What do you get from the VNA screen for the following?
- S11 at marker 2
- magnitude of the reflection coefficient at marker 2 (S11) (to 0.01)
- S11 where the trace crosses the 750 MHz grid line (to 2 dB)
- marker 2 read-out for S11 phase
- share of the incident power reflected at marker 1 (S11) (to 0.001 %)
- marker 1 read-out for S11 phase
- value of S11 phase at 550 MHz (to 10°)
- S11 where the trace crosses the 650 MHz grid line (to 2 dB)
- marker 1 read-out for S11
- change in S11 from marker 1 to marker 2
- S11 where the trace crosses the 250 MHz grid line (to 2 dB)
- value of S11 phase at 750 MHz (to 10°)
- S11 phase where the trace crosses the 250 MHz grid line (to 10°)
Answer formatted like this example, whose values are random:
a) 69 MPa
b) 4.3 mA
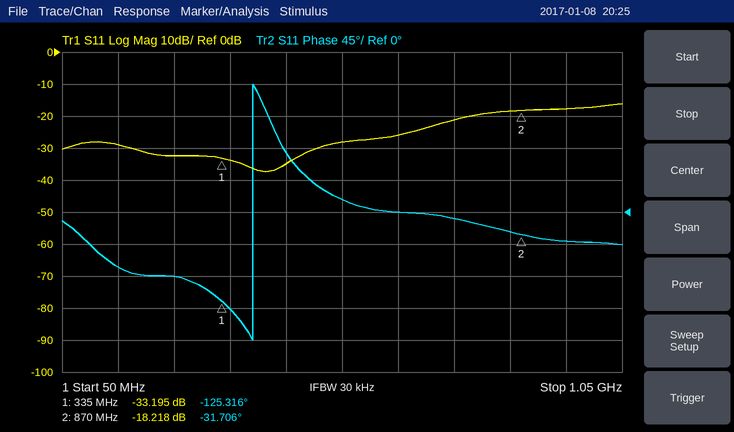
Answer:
a) -18.218 dB
b) 0.12
c) -22 dB
d) -31.706°
e) 0.048 %
f) -125.316°
g) 20°
h) -26 dB
i) -33.195 dB
j) 14.977 dB
k) -32 dB
l) -10°
m) -90°
